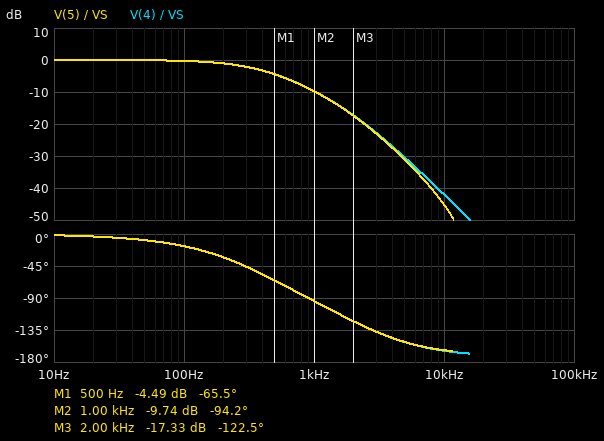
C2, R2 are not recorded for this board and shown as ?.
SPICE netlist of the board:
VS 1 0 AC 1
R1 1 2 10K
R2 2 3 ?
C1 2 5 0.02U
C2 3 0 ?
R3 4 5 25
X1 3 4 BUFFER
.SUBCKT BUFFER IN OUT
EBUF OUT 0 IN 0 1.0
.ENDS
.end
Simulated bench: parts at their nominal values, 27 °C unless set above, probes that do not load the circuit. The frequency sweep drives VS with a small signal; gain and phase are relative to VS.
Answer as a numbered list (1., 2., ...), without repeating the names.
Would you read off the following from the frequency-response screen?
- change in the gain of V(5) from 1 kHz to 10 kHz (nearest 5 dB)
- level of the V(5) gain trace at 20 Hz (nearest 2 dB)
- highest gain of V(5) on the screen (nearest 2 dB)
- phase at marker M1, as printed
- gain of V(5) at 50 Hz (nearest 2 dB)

1. -35 dB
2. 0 dB
3. 0 dB
4. -65.5 deg
5. 0 dB
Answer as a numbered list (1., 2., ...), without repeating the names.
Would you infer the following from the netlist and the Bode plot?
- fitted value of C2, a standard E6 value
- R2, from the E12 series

1. 33 nF
2. 4.7 kΩ
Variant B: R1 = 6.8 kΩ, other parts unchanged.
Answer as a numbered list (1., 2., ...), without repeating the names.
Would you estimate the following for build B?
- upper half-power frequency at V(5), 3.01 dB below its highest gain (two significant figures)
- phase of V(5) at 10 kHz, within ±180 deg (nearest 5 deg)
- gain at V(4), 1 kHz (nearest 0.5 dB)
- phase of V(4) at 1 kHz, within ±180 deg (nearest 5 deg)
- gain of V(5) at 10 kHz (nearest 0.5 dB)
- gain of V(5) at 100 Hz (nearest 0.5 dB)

1. 490 Hz
2. -160 deg
3. -7.5 dB
4. -85 deg
5. -42.0 dB
6. 0 dB
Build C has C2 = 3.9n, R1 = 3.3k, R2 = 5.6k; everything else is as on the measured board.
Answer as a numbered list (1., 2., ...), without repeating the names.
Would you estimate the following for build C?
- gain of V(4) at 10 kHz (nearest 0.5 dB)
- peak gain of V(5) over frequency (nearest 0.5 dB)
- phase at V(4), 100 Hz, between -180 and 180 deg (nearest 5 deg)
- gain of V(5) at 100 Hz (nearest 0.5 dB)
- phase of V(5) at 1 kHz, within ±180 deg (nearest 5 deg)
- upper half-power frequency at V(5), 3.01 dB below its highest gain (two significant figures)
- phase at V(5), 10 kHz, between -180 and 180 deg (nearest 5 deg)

1. -14.5 dB
2. 1.5 dB
3. 0 deg
4. 0 dB
5. -15 deg
6. 4.9 kHz
7. -155 deg
